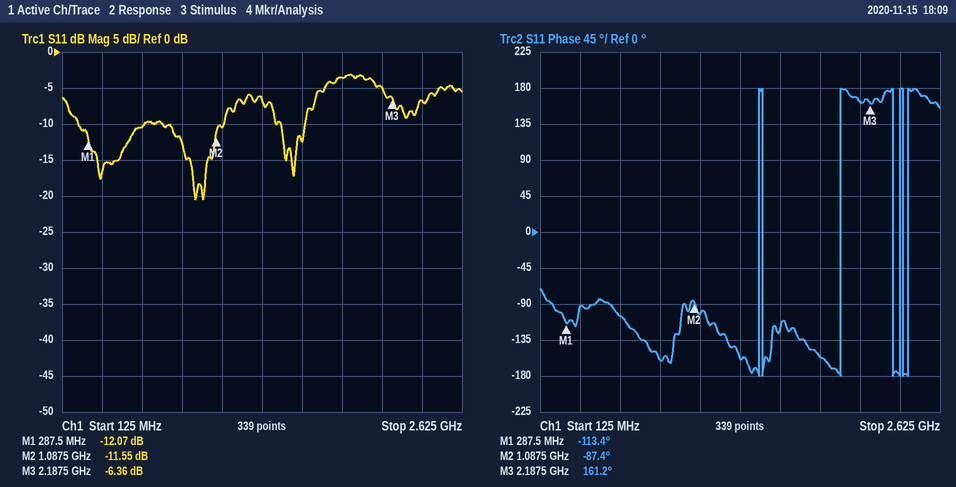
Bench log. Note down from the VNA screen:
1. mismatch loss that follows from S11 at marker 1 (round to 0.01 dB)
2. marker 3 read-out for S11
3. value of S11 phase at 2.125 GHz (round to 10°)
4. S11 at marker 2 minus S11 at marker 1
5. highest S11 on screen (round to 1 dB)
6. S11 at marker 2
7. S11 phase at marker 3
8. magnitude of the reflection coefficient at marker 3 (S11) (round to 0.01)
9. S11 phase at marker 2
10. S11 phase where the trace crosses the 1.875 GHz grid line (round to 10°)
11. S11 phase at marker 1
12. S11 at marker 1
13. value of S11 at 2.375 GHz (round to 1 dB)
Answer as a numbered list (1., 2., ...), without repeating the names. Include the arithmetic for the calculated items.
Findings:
1. −10 log10(1 − 10^(-12.07/10)) ≈ 0.28 dB
2. -6.36 dB
3. 160°
4. -11.55 − (-12.07) = 0.52 dB
5. -3 dB
6. -11.55 dB
7. 161.2°
8. 10^(-6.36/20) ≈ 0.48
9. -87.4°
10. -160°
11. -113.4°
12. -12.07 dB
13. -7 dB
